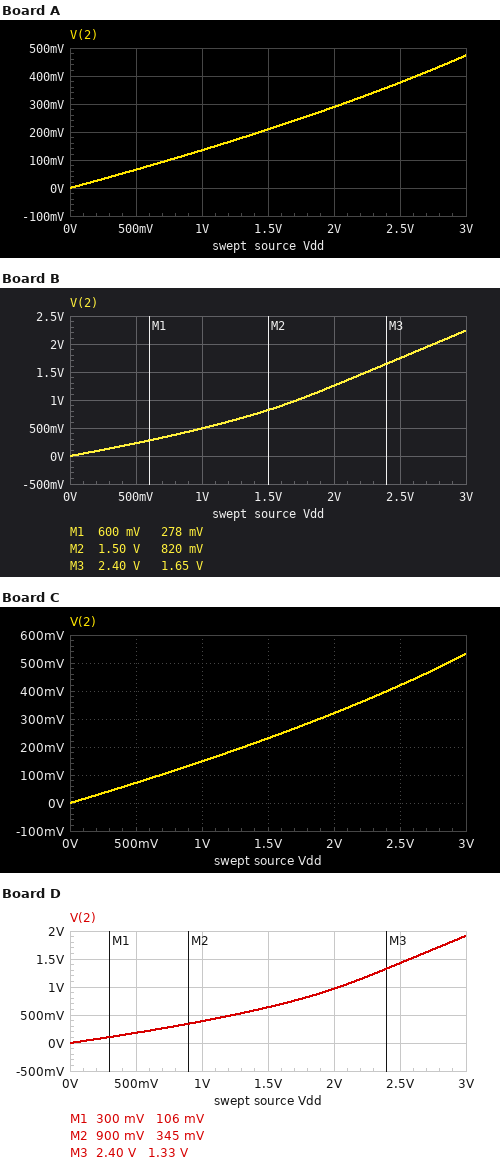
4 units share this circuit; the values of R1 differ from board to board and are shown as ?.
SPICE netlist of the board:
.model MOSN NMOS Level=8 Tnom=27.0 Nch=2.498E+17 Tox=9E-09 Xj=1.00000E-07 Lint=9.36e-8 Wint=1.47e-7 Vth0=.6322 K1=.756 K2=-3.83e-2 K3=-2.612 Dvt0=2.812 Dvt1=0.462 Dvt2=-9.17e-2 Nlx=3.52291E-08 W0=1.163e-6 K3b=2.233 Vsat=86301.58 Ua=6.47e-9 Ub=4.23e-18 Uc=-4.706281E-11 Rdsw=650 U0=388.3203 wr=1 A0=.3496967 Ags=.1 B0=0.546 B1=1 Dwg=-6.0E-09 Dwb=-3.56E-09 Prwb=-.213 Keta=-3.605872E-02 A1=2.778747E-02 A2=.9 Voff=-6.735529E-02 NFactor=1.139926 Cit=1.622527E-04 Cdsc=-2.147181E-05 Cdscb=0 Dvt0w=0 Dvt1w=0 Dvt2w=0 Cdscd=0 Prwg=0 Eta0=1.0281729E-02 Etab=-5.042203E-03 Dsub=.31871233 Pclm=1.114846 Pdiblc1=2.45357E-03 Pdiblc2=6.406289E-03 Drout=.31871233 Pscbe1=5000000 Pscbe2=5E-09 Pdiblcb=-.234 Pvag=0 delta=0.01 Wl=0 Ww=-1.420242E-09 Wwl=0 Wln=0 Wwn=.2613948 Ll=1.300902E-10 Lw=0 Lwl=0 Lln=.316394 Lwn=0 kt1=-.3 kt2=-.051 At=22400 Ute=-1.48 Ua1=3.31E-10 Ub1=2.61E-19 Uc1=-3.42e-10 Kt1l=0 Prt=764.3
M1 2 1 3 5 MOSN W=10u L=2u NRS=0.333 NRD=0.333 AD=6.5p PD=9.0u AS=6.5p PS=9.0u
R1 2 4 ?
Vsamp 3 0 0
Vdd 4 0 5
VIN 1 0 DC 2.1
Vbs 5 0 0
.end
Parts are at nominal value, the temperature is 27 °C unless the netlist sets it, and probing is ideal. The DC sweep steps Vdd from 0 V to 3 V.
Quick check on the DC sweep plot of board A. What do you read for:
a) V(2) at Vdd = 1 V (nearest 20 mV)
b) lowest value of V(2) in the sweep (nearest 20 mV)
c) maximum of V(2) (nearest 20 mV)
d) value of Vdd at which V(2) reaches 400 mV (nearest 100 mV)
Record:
140 mV
0 V
480 mV
2.6 V
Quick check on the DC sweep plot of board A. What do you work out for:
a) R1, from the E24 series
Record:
20 kΩ
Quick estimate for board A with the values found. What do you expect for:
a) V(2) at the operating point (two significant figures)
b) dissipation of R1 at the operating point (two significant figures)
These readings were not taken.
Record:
1.2 V
720 µW
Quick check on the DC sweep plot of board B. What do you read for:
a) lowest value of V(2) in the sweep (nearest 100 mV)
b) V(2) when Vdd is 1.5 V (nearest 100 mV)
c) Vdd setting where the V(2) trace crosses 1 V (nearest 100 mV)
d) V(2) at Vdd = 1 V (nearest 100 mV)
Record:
0 V
800 mV
1.7 V
500 mV
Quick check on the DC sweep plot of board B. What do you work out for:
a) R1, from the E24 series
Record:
3.9 kΩ
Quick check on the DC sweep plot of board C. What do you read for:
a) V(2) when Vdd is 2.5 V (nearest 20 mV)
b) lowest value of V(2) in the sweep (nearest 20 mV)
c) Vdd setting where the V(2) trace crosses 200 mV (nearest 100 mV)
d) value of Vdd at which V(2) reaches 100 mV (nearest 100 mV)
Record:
420 mV
0 V
1.3 V
700 mV
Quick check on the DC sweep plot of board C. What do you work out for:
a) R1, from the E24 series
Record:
18 kΩ
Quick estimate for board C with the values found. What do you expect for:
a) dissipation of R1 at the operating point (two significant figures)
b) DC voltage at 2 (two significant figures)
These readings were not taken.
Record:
670 µW
1.5 V
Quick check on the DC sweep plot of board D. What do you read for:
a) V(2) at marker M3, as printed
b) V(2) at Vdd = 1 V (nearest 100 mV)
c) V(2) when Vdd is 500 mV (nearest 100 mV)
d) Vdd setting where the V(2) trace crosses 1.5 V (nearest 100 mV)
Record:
1.33 V
400 mV
200 mV
2.6 V
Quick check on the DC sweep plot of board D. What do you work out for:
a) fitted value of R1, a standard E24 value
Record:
5.6 kΩ
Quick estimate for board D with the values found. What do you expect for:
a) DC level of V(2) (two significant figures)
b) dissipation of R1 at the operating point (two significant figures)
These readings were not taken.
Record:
3.9 V
220 µW
